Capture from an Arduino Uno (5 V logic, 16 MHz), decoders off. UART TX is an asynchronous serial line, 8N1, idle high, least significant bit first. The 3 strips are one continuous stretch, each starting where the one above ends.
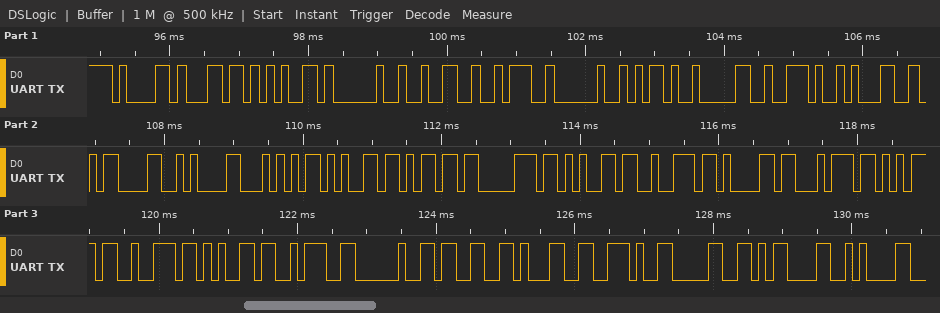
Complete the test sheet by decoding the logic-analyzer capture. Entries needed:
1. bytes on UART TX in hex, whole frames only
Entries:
0x61 0x6C 0x65 0x20 0x32 0x3A 0x20 0x2D 0x30 0x2E 0x31 0x0D 0x0A 0x54 0x65 0x6D 0x70 0x65 0x72 0x61 0x74 0x75 0x72 0x65 0x3A 0x20 0x33 0x31 0x2E 0x30 0x0D 0x0A
